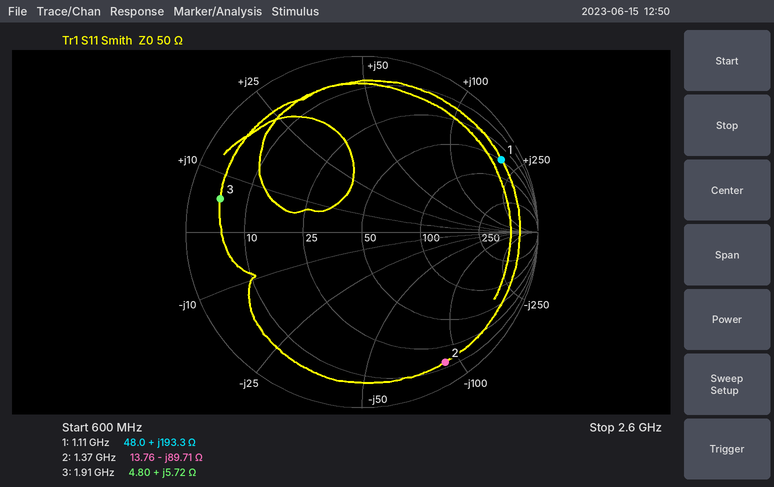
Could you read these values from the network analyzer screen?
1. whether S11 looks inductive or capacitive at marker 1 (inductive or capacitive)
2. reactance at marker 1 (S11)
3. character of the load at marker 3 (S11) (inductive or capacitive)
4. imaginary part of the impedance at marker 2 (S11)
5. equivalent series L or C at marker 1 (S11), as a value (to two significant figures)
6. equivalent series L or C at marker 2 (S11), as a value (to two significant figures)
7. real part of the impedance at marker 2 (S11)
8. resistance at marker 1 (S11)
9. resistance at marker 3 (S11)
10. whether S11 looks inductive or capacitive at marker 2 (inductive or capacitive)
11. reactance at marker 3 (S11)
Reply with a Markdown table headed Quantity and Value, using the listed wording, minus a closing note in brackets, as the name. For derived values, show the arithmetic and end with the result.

| Quantity | Value |
|---|---|
| whether S11 looks inductive or capacitive at marker 1 | inductive |
| reactance at marker 1 | +193.3 Ω |
| character of the load at marker 3 (S11) | inductive |
| imaginary part of the impedance at marker 2 | -89.71 Ω |
| equivalent series L or C at marker 1 (S11), as a value | L = 193.3 Ω/(2π × 1.11 GHz) ≈ 28 nH |
| equivalent series L or C at marker 2 (S11), as a value | C = 1/(2π × 1.37 GHz × 89.71 Ω) ≈ 1.3 pF |
| real part of the impedance at marker 2 | 13.76 Ω |
| resistance at marker 1 | 48.0 Ω |
| resistance at marker 3 | 4.80 Ω |
| whether S11 looks inductive or capacitive at marker 2 | capacitive |
| reactance at marker 3 | +5.72 Ω |
